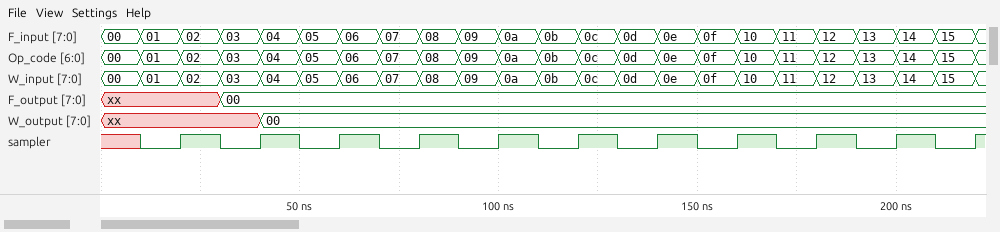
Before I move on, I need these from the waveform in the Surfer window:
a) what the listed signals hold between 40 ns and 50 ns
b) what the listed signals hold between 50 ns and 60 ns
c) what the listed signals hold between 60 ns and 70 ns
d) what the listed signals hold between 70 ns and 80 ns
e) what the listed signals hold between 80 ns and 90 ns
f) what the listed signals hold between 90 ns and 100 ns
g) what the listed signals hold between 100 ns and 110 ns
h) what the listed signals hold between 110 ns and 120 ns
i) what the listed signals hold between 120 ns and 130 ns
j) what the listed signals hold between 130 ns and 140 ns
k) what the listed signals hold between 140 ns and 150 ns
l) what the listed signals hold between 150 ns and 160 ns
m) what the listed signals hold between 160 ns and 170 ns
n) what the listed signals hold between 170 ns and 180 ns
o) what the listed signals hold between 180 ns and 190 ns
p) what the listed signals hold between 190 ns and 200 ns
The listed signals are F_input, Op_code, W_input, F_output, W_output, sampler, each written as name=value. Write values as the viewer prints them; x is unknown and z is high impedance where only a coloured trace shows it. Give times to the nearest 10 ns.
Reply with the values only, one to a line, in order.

F_input=04, Op_code=04, W_input=04, F_output=00, W_output=00, sampler=1
F_input=05, Op_code=05, W_input=05, F_output=00, W_output=00, sampler=0
F_input=06, Op_code=06, W_input=06, F_output=00, W_output=00, sampler=1
F_input=07, Op_code=07, W_input=07, F_output=00, W_output=00, sampler=0
F_input=08, Op_code=08, W_input=08, F_output=00, W_output=00, sampler=1
F_input=09, Op_code=09, W_input=09, F_output=00, W_output=00, sampler=0
F_input=0a, Op_code=0a, W_input=0a, F_output=00, W_output=00, sampler=1
F_input=0b, Op_code=0b, W_input=0b, F_output=00, W_output=00, sampler=0
F_input=0c, Op_code=0c, W_input=0c, F_output=00, W_output=00, sampler=1
F_input=0d, Op_code=0d, W_input=0d, F_output=00, W_output=00, sampler=0
F_input=0e, Op_code=0e, W_input=0e, F_output=00, W_output=00, sampler=1
F_input=0f, Op_code=0f, W_input=0f, F_output=00, W_output=00, sampler=0
F_input=10, Op_code=10, W_input=10, F_output=00, W_output=00, sampler=1
F_input=11, Op_code=11, W_input=11, F_output=00, W_output=00, sampler=0
F_input=12, Op_code=12, W_input=12, F_output=00, W_output=00, sampler=1
F_input=13, Op_code=13, W_input=13, F_output=00, W_output=00, sampler=0
